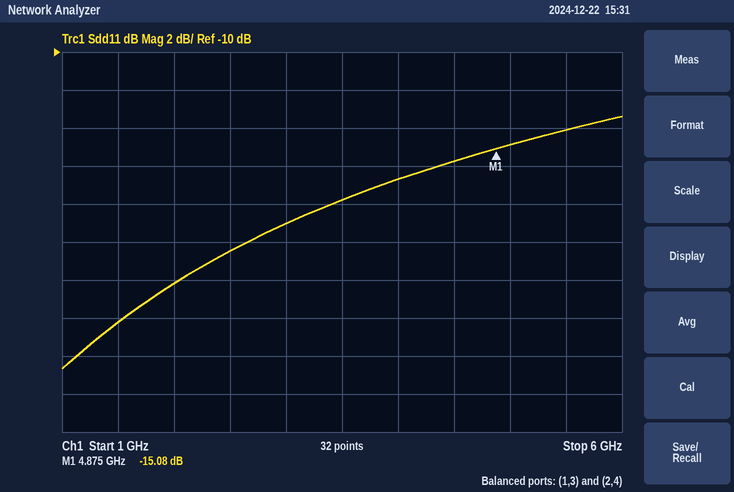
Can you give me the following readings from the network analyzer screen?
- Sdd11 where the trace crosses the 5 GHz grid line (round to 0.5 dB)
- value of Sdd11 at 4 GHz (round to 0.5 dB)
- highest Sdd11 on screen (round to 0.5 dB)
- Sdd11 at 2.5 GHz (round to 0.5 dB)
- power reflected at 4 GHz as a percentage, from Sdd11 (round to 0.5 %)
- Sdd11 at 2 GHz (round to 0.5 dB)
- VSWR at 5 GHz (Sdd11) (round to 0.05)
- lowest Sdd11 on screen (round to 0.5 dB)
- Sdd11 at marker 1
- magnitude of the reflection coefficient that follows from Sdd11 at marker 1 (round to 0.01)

-15.0 dB
-16.5 dB
-13.5 dB
-20.5 dB
2.0 %
-22.0 dB
1.45
-26.5 dB
-15.08 dB
0.18
